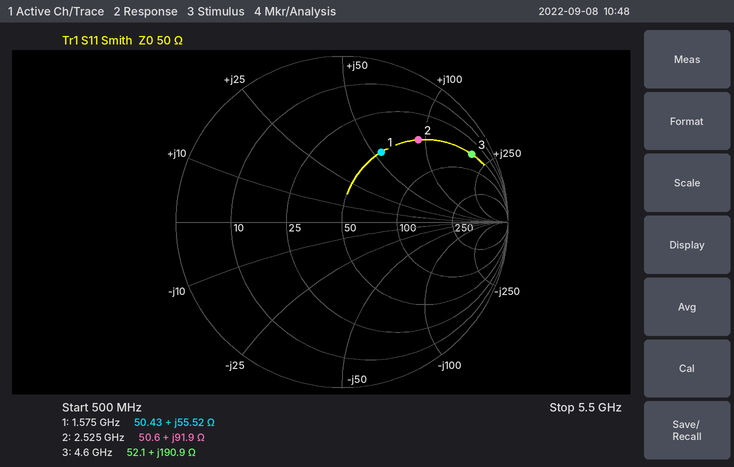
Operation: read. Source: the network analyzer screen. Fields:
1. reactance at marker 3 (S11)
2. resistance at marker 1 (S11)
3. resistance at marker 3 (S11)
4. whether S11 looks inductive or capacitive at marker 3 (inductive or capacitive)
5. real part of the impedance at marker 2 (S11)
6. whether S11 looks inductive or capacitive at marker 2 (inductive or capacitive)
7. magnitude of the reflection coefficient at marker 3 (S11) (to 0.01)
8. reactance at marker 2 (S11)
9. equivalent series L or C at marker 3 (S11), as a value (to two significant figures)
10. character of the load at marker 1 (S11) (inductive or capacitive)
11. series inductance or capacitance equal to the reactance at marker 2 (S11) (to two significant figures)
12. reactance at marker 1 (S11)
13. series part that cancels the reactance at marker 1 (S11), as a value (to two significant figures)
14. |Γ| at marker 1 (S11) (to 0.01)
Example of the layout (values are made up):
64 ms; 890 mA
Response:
+190.9 Ω; 50.43 Ω; 52.1 Ω; inductive; 50.6 Ω; inductive; 0.88; +91.9 Ω; 6.6 nH; inductive; 5.8 nH; +55.52 Ω; 1.8 pF; 0.48
